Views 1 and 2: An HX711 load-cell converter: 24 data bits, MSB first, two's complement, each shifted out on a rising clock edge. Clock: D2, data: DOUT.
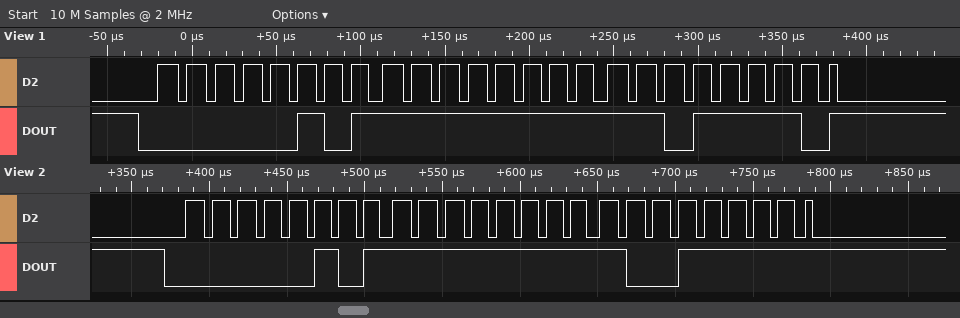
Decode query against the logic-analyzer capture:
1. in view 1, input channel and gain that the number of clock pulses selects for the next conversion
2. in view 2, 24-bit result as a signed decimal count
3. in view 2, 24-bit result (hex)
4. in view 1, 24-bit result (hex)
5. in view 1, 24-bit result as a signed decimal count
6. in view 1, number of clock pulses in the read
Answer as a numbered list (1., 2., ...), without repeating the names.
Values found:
1. channel A, gain 128
2. 393119
3. 0x05FF9F
4. 0x05FFDE
5. 393182
6. 25
